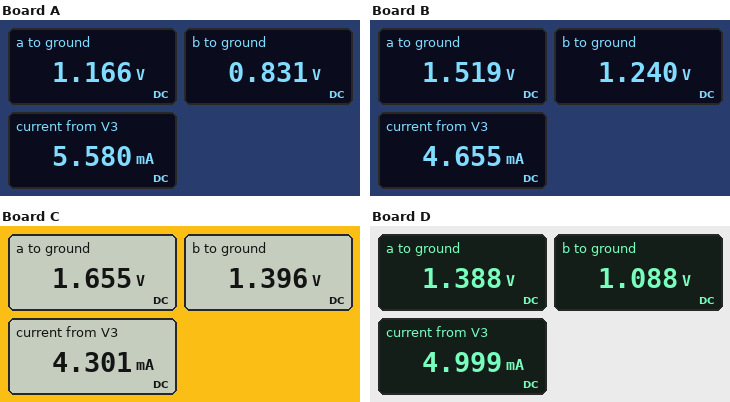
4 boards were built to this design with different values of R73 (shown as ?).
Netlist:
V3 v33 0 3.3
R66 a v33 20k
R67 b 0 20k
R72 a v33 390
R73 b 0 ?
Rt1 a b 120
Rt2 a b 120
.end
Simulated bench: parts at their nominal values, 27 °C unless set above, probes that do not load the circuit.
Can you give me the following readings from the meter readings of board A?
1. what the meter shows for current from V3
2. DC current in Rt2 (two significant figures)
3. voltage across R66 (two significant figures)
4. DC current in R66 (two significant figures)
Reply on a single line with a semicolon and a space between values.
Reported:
5.580 mA; 2.8 mA; 2.1 V; 110 µA
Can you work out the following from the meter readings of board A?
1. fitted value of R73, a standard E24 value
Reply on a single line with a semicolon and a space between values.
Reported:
150 Ω
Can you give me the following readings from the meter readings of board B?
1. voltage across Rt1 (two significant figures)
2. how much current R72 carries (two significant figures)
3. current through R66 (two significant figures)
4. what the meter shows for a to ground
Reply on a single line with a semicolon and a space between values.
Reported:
280 mV; 4.6 mA; 89 µA; 1.519 V
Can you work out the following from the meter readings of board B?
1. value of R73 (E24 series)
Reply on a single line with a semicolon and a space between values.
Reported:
270 Ω
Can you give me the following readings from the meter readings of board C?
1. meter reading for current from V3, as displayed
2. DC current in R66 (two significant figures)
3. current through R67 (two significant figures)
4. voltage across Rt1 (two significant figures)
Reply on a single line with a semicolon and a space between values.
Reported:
4.301 mA; 82 µA; 70 µA; 260 mV
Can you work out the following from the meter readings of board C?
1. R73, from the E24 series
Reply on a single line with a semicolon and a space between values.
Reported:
330 Ω
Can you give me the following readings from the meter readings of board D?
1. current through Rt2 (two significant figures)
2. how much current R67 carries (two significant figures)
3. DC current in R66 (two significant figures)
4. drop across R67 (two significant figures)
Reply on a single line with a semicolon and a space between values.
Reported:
2.5 mA; 54 µA; 96 µA; 1.1 V
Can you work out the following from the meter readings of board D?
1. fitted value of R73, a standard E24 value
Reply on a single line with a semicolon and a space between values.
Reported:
220 Ω
